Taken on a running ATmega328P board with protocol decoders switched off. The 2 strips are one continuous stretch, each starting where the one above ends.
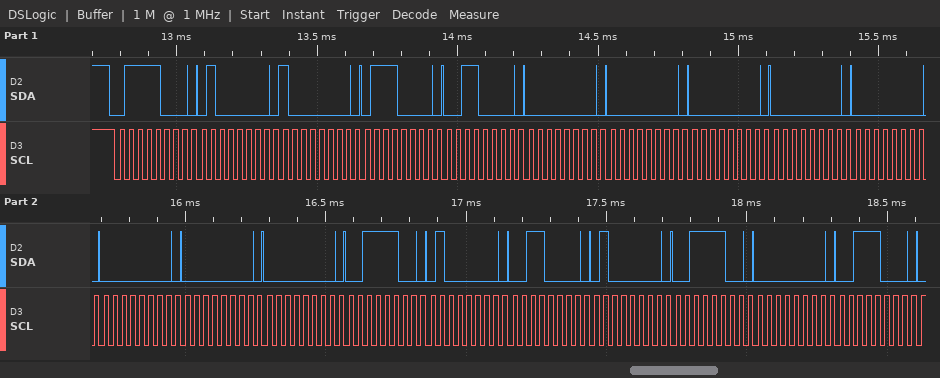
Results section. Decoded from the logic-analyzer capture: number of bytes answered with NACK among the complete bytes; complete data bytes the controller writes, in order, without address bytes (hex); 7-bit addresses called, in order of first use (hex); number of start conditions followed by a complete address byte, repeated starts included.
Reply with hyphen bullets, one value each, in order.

- 0
- 40 80 70 30 00 00 00 00 00 00 00 00 3C 40 30 40 3C 00 38
- 0x3C
- 1
